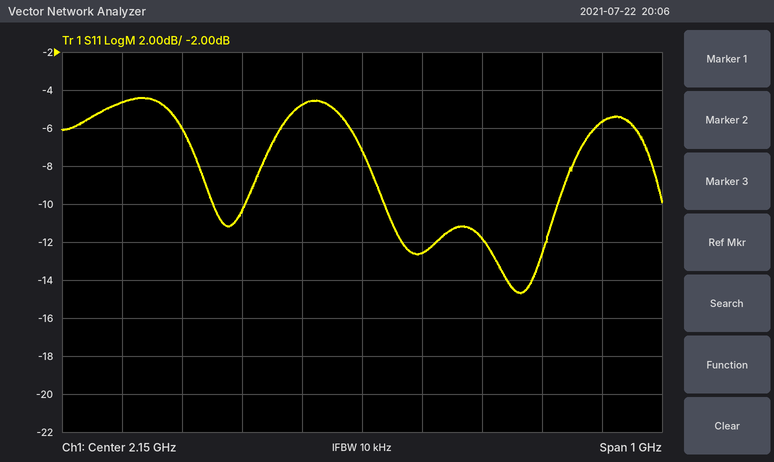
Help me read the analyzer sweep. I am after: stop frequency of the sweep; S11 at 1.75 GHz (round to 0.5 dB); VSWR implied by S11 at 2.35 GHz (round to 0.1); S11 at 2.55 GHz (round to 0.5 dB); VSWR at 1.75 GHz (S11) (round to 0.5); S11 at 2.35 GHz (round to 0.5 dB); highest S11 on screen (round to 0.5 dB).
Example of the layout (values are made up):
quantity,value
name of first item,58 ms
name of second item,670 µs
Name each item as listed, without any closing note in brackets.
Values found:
quantity,value
stop frequency of the sweep,2.65 GHz
S11 at 1.75 GHz,-4.5 dB
VSWR implied by S11 at 2.35 GHz,1.7
S11 at 2.55 GHz,-5.5 dB
VSWR at 1.75 GHz (S11),4.0
S11 at 2.35 GHz,-12.0 dB
highest S11 on screen,-4.5 dB
